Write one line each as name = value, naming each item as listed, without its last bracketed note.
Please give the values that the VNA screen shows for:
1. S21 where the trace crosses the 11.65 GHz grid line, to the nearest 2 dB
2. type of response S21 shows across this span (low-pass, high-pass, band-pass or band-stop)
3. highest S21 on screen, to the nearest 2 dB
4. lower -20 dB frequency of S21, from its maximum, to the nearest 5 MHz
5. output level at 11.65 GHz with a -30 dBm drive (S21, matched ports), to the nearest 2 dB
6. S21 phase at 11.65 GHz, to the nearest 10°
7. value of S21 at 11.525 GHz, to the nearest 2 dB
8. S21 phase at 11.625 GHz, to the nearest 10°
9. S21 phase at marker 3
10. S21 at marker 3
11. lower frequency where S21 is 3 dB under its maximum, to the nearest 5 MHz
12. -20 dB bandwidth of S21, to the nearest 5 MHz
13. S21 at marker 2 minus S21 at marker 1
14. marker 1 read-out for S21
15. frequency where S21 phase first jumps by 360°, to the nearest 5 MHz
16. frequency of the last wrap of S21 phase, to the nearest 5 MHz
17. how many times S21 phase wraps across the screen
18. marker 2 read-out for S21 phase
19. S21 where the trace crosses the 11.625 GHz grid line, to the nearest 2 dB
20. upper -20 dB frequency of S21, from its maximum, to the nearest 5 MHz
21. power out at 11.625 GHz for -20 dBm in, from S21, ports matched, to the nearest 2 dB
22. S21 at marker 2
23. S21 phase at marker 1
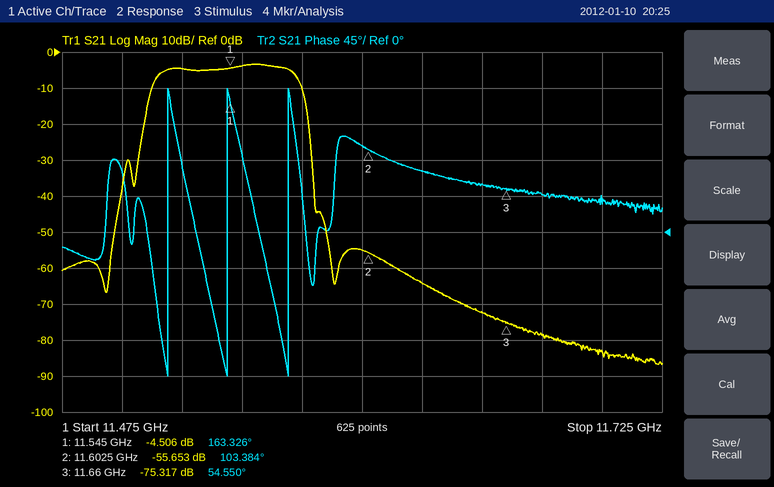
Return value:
S21 where the trace crosses the 11.65 GHz grid line, to the nearest 2 dB = -72 dB
type of response S21 shows across this span = band-pass
highest S21 on screen, to the nearest 2 dB = -4 dB
lower -20 dB frequency of S21, from its maximum, to the nearest 5 MHz = 11.510 GHz
output level at 11.65 GHz with a -30 dBm drive (S21, matched ports), to the nearest 2 dB = -102 dBm
S21 phase at 11.65 GHz, to the nearest 10° = 60°
value of S21 at 11.525 GHz, to the nearest 2 dB = -4 dB
S21 phase at 11.625 GHz, to the nearest 10° = 80°
S21 phase at marker 3 = 54.550°
S21 at marker 3 = -75.317 dB
lower frequency where S21 is 3 dB under its maximum, to the nearest 5 MHz = 11.515 GHz
-20 dB bandwidth of S21, to the nearest 5 MHz = 70 MHz
S21 at marker 2 minus S21 at marker 1 = -51.147 dB
marker 1 read-out for S21 = -4.506 dB
frequency where S21 phase first jumps by 360°, to the nearest 5 MHz = 11.520 GHz
frequency of the last wrap of S21 phase, to the nearest 5 MHz = 11.570 GHz
how many times S21 phase wraps across the screen = 3
marker 2 read-out for S21 phase = 103.384°
S21 where the trace crosses the 11.625 GHz grid line, to the nearest 2 dB = -64 dB
upper -20 dB frequency of S21, from its maximum, to the nearest 5 MHz = 11.580 GHz
power out at 11.625 GHz for -20 dBm in, from S21, ports matched, to the nearest 2 dB = -84 dBm
S21 at marker 2 = -55.653 dB
S21 phase at marker 1 = 163.326°
